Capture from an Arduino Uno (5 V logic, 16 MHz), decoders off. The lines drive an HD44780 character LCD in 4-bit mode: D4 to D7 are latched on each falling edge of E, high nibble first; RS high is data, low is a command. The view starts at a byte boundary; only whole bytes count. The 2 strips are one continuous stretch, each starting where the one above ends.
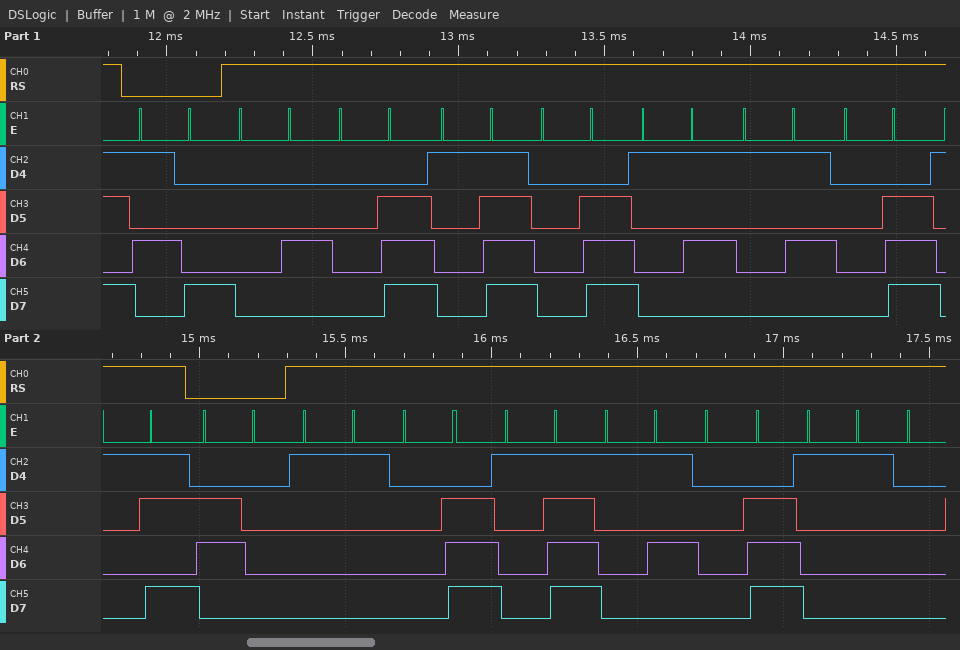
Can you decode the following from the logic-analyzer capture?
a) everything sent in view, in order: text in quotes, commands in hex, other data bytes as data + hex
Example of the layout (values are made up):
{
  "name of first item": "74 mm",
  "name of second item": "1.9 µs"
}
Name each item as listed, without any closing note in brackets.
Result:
{
  "everything sent in view, in order: text in quotes, commands in hex, other data bytes as data + hex": "0x58 data 04 0E 1F 0E 15 15 0E 1B 0x60 data 11 0E 1F 15 0E 11"
}
